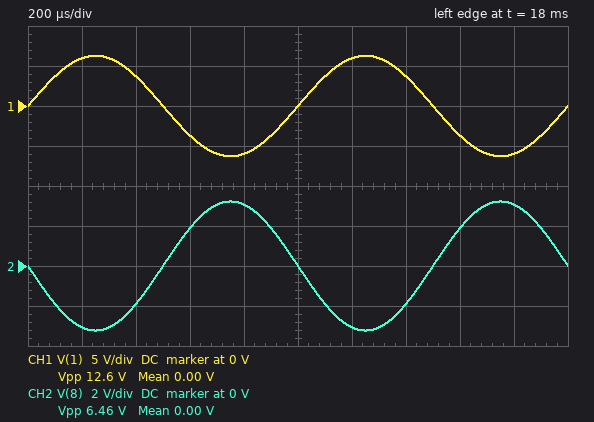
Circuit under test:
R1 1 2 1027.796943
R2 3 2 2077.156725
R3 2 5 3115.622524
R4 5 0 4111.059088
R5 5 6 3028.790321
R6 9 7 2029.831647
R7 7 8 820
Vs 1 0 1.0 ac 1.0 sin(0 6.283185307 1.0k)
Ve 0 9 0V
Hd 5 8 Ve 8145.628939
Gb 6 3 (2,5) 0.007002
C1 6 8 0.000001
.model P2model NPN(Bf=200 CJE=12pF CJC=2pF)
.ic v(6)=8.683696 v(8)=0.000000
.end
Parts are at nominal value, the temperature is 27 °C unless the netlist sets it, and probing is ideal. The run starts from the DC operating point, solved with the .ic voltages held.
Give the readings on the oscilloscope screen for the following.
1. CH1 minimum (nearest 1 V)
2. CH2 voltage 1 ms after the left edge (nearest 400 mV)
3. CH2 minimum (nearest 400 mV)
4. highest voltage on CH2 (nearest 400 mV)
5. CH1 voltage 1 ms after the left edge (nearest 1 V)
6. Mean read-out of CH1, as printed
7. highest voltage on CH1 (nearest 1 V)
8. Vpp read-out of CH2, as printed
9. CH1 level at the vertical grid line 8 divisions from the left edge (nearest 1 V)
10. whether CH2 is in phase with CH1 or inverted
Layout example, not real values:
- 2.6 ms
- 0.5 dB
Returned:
- -6 V
- 0 V
- -3.2 V
- 3.2 V
- 0 V
- 0.00 V
- 6 V
- 6.46 V
- -4 V
- inverted
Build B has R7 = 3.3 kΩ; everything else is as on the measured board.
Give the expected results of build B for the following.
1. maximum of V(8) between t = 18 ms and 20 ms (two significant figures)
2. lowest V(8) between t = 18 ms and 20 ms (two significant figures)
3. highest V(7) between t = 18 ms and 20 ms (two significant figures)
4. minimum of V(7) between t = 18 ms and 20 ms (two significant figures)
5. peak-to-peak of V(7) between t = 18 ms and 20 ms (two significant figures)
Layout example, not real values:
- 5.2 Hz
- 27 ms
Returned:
- 13 V
- -13 V
- 5.0 V
- -5.0 V
- 10 V
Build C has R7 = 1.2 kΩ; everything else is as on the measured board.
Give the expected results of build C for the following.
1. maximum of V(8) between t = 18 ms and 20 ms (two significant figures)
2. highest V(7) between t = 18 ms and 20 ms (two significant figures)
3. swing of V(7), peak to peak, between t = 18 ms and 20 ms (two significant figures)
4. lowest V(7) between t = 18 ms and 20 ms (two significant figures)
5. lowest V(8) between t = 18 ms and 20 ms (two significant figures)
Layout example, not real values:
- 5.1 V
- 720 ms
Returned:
- 4.0 V
- 2.5 V
- 5.0 V
- -2.5 V
- -4.0 V
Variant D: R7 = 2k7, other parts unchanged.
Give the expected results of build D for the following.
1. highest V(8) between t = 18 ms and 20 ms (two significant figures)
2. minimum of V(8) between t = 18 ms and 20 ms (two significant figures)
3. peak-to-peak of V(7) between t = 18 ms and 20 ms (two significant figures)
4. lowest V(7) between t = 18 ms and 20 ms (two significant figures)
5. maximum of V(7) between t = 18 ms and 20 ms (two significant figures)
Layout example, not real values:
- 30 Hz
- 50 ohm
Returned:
- 9.1 V
- -9.1 V
- 7.8 V
- -3.9 V
- 3.9 V
